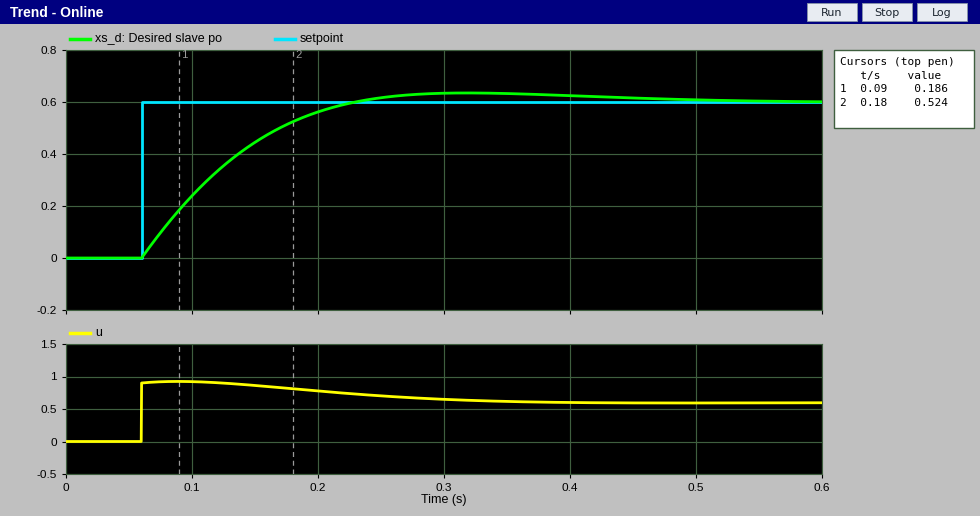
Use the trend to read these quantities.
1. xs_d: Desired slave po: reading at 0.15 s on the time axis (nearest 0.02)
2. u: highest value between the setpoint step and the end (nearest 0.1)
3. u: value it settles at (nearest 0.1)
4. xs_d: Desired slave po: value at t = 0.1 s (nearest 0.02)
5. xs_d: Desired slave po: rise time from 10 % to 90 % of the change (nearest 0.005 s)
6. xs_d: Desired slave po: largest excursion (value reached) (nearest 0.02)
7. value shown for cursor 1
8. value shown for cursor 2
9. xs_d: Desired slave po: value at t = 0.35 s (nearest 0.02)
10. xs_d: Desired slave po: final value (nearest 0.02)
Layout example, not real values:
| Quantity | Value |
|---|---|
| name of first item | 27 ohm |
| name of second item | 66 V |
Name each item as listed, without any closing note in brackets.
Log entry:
| Quantity | Value |
|---|---|
| xs_d: Desired slave po: reading at 0.15 s on the time axis | 0.44 |
| u: highest value between the setpoint step and the end | 0.9 |
| u: value it settles at | 0.6 |
| xs_d: Desired slave po: value at t = 0.1 s | 0.24 |
| xs_d: Desired slave po: rise time from 10 % to 90 % of the change | 0.120 s |
| xs_d: Desired slave po: largest excursion (value reached) | 0.64 |
| value shown for cursor 1 | 0.186 |
| value shown for cursor 2 | 0.524 |
| xs_d: Desired slave po: value at t = 0.35 s | 0.64 |
| xs_d: Desired slave po: final value | 0.60 |
